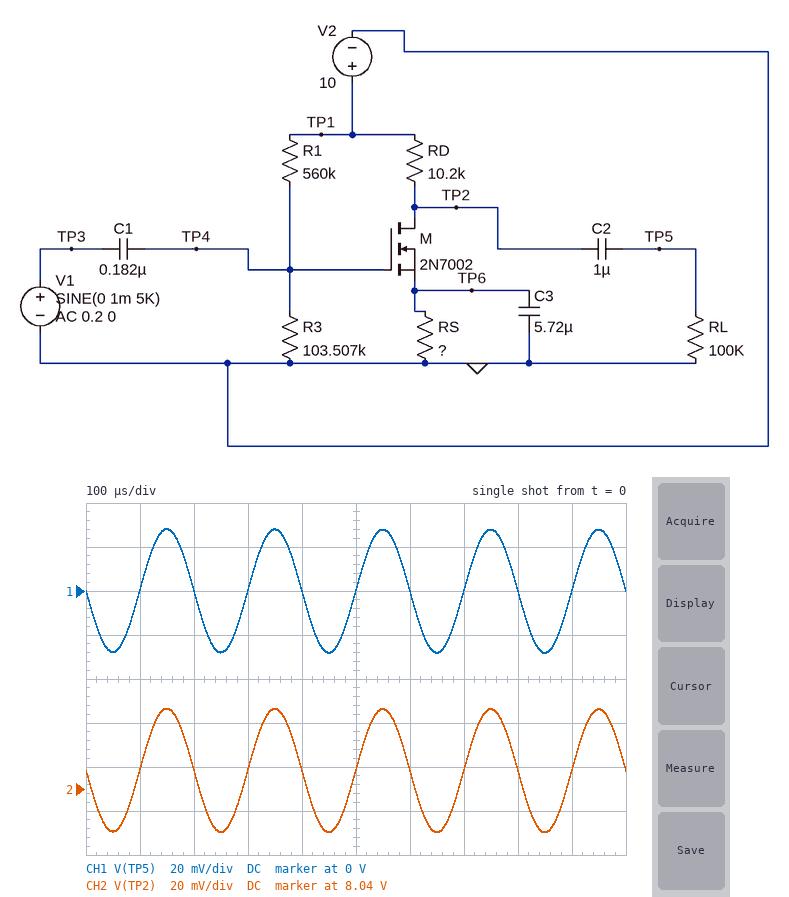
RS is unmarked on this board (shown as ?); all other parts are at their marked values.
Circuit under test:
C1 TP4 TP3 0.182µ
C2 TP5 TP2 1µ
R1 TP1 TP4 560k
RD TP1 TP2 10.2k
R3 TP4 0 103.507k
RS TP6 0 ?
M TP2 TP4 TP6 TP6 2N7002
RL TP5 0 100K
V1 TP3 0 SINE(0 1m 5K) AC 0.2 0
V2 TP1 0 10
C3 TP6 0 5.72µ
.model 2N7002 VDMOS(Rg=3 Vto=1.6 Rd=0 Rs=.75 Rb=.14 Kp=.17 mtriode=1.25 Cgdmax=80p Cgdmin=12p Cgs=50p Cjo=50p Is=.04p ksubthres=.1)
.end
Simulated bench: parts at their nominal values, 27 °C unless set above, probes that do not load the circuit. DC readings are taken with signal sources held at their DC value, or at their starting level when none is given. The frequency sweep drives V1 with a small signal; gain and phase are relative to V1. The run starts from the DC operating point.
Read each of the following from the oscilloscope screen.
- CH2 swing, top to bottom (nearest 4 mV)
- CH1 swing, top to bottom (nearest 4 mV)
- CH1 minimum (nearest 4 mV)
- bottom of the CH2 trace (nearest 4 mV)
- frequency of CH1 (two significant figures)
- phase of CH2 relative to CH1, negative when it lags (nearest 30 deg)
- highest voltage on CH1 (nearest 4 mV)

56 mV
56 mV
-28 mV
8.020 V
5.0 kHz
0 deg
28 mV
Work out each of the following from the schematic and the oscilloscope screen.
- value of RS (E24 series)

51 Ω
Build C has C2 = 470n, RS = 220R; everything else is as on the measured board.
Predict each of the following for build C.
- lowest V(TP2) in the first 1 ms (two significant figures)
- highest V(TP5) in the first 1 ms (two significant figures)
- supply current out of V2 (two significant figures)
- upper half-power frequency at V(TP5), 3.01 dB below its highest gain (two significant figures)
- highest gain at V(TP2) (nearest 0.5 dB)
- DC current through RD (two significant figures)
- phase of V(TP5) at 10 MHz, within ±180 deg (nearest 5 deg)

8.6 V
21 mV
150 µA
570 kHz
26.5 dB
140 µA
70 deg
